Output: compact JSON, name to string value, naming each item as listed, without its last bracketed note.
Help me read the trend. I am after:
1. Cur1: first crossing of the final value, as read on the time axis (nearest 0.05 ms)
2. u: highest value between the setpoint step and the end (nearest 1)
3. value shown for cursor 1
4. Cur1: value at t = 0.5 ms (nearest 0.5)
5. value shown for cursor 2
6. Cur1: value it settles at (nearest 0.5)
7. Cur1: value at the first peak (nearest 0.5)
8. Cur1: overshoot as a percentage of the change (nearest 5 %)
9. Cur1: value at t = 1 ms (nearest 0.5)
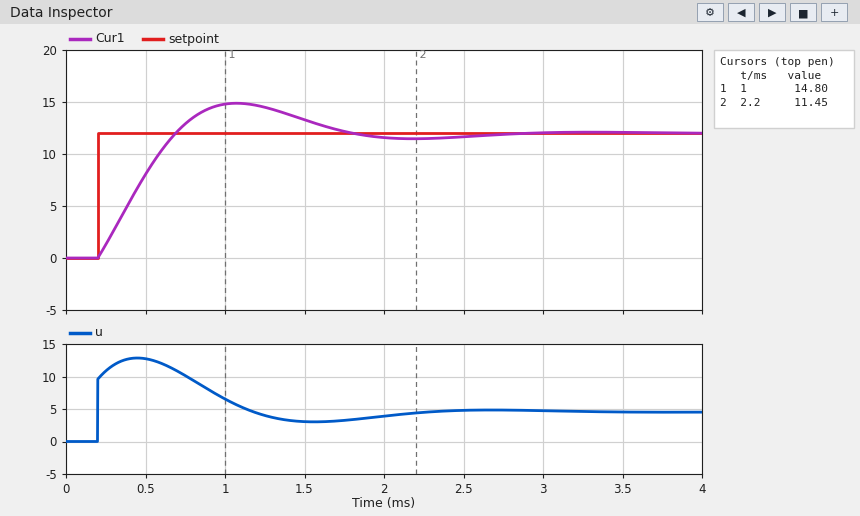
{"Cur1: first crossing of the final value, as read on the time axis": "0.70 ms", "u: highest value between the setpoint step and the end": "13", "value shown for cursor 1": "14.80", "Cur1: value at t = 0.5 ms": "8.0", "value shown for cursor 2": "11.45", "Cur1: value it settles at": "12.0", "Cur1: value at the first peak": "15.0", "Cur1: overshoot as a percentage of the change": "25 %", "Cur1: value at t = 1 ms": "15.0"}
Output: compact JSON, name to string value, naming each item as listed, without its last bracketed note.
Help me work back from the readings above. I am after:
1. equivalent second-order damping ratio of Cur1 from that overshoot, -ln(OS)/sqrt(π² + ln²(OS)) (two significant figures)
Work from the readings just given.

{"equivalent second-order damping ratio of Cur1 from that overshoot, -ln(OS)/sqrt(π² + ln²(OS))": "0.40"}
